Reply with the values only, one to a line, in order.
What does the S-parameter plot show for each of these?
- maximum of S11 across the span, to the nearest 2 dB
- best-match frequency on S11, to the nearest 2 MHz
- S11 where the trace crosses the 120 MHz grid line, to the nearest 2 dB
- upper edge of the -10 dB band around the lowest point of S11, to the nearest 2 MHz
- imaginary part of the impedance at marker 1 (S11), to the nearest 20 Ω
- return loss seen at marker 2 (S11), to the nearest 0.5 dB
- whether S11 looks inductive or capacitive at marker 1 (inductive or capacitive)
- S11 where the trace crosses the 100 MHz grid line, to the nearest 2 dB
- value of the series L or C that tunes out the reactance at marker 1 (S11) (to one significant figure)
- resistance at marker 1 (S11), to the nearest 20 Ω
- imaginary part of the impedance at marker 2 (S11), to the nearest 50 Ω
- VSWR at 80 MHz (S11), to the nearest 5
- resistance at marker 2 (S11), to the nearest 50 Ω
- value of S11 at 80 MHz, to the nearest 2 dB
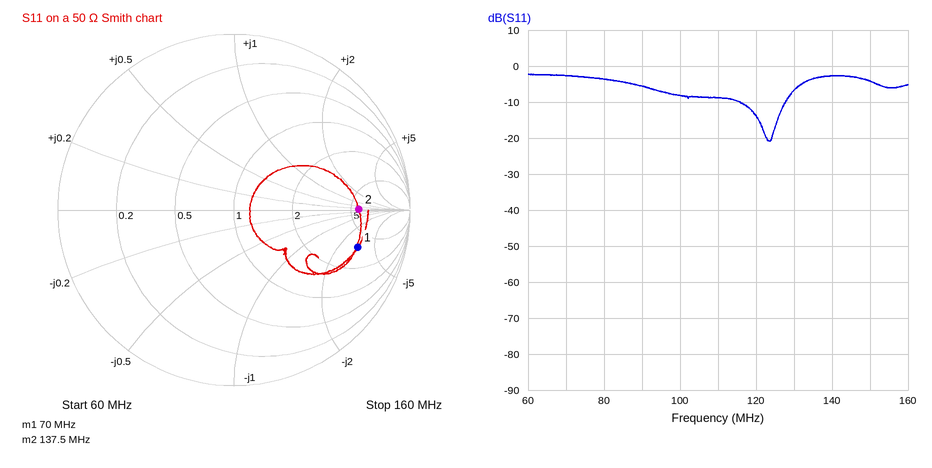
-2 dB
124 MHz
-14 dB
128 MHz
-160 Ω
3.0 dB
capacitive
-8 dB
400 nH
180 Ω
0 Ω
5
300 Ω
-4 dB
